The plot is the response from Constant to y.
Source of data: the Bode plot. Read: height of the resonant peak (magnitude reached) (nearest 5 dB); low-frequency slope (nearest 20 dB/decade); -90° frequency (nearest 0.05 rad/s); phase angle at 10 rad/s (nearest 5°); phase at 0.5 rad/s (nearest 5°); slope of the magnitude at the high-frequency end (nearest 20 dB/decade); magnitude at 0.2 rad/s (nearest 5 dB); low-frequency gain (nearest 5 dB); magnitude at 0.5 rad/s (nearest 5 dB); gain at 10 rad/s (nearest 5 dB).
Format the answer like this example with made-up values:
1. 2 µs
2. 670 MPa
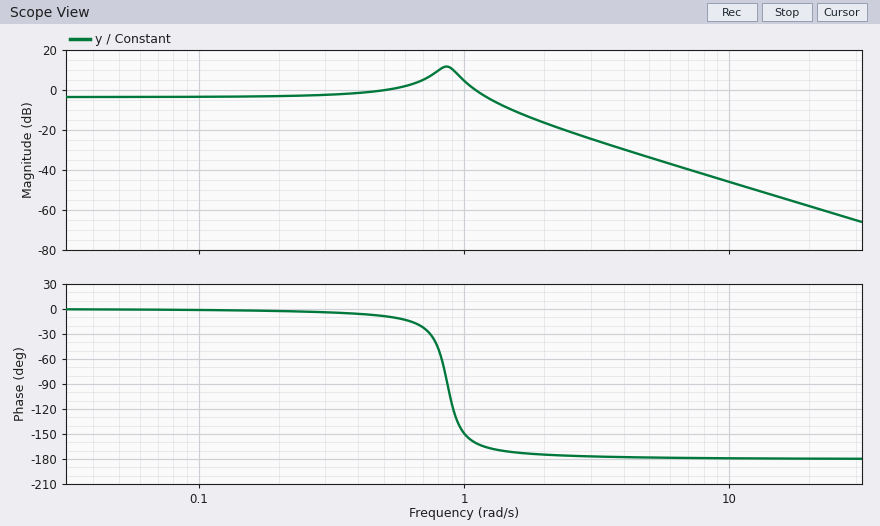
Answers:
1. 10 dB
2. 0 dB/decade
3. 0.85 rad/s
4. -180°
5. -10°
6. -40 dB/decade
7. -5 dB
8. -5 dB
9. 0 dB
10. -45 dB
